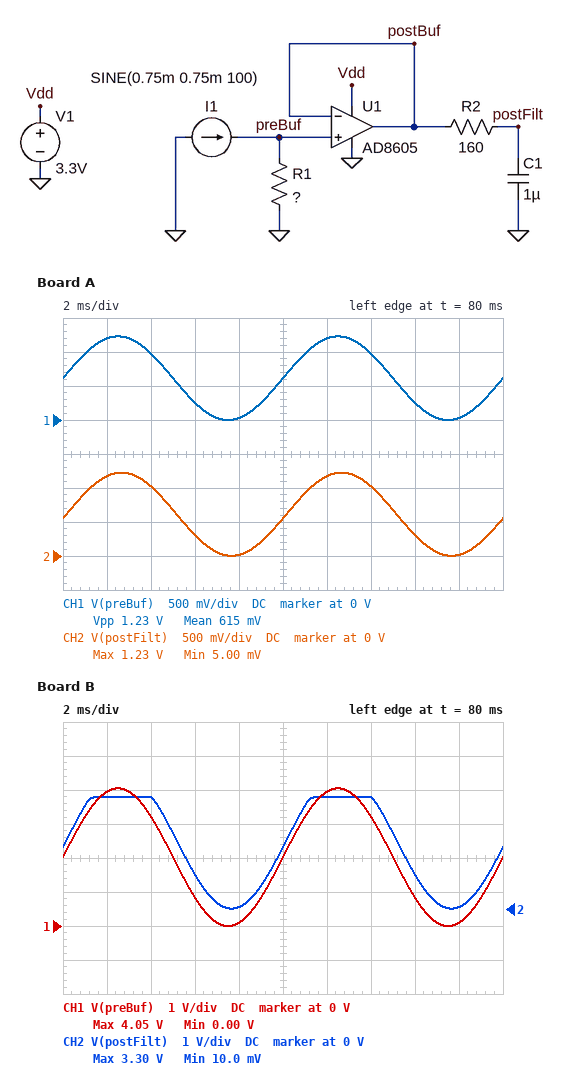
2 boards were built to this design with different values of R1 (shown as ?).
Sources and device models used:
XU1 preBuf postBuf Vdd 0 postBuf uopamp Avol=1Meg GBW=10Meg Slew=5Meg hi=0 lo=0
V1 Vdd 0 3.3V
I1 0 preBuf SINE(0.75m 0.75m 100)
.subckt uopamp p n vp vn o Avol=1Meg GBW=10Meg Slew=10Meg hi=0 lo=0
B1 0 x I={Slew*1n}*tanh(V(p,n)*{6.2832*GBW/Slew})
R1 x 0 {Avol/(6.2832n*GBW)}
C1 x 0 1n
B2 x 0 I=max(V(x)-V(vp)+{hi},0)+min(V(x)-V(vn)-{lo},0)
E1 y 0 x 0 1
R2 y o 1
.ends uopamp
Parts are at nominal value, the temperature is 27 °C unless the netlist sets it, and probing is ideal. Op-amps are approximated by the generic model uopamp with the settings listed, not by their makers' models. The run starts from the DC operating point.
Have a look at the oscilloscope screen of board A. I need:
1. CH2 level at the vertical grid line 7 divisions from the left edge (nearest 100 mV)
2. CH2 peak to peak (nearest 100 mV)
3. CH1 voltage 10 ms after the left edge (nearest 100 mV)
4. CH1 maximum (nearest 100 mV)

1.0 V
1.2 V
600 mV
1.2 V
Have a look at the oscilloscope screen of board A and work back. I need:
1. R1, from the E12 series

820 Ω
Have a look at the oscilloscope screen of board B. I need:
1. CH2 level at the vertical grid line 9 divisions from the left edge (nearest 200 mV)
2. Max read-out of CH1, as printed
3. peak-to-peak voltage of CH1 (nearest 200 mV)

0 V
4.05 V
4.0 V
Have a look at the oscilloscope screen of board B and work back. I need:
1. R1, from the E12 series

2.7 kΩ
